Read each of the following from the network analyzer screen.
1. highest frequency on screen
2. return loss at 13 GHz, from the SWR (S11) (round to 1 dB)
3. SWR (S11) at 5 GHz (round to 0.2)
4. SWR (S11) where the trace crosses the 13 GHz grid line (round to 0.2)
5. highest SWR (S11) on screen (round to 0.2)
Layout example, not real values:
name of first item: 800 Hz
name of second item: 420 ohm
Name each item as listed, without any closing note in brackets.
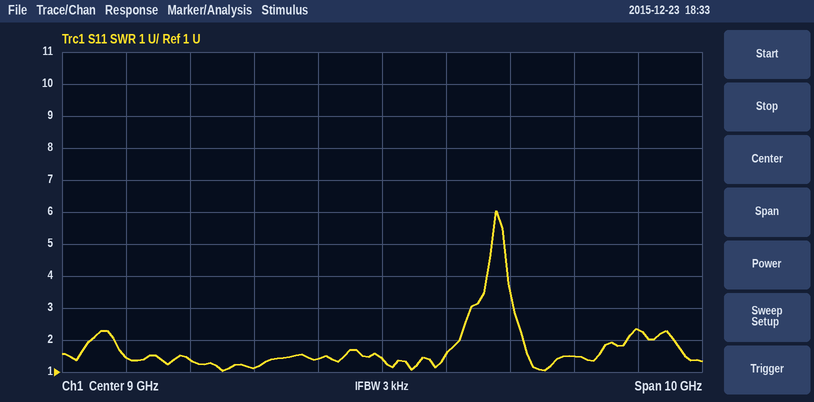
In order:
highest frequency on screen: 14 GHz
return loss at 13 GHz, from the SWR (S11): 8 dB
SWR (S11) at 5 GHz: 1.4
SWR (S11) where the trace crosses the 13 GHz grid line: 2.4
highest SWR (S11) on screen: 6.0
